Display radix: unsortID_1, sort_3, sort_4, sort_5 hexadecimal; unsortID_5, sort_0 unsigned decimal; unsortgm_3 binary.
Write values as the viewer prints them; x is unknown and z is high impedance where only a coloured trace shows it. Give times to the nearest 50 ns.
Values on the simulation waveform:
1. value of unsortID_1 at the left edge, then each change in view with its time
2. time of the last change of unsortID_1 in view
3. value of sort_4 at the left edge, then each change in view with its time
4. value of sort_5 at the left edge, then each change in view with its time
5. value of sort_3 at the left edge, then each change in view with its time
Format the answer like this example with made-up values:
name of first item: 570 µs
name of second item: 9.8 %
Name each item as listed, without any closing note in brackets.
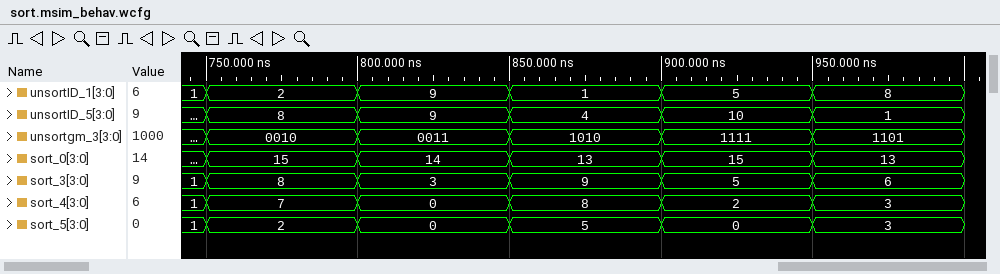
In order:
value of unsortID_1 at the left edge, then each change in view with its time: 1, 2 at 750 ns, 9 at 800 ns, 1 at 850 ns, 5 at 900 ns, 8 at 950 ns
time of the last change of unsortID_1 in view: 950 ns
value of sort_4 at the left edge, then each change in view with its time: 1, 7 at 750 ns, 0 at 800 ns, 8 at 850 ns, 2 at 900 ns, 3 at 950 ns
value of sort_5 at the left edge, then each change in view with its time: 1, 2 at 750 ns, 0 at 800 ns, 5 at 850 ns, 0 at 900 ns, 3 at 950 ns
value of sort_3 at the left edge, then each change in view with its time: 1, 8 at 750 ns, 3 at 800 ns, 9 at 850 ns, 5 at 900 ns, 6 at 950 ns
